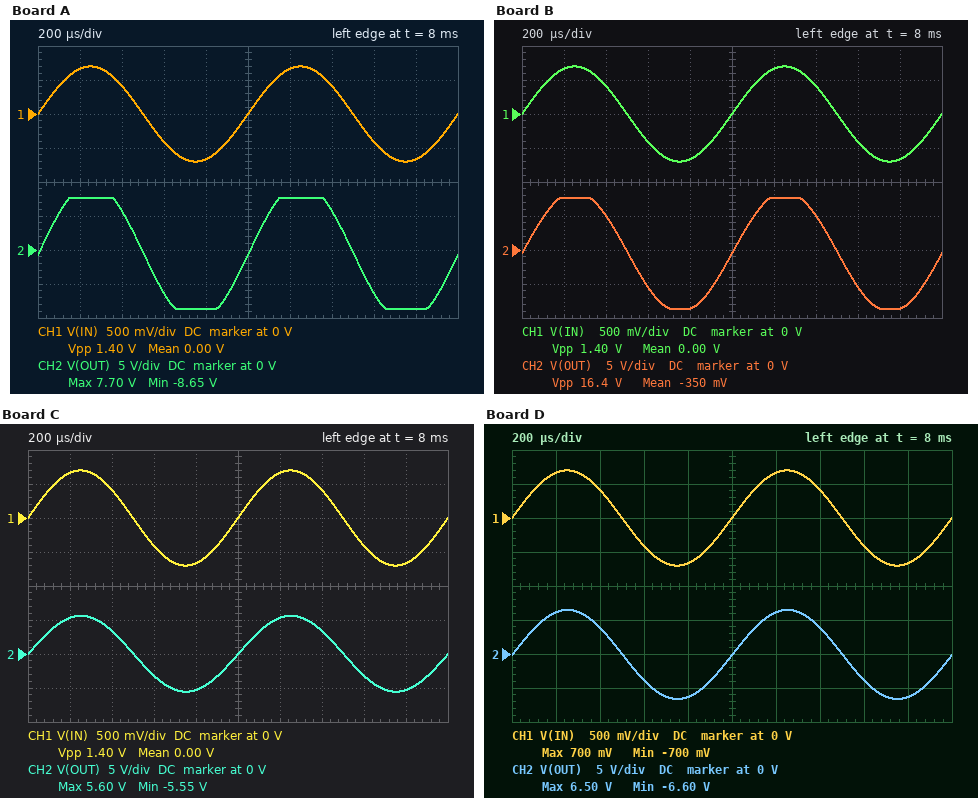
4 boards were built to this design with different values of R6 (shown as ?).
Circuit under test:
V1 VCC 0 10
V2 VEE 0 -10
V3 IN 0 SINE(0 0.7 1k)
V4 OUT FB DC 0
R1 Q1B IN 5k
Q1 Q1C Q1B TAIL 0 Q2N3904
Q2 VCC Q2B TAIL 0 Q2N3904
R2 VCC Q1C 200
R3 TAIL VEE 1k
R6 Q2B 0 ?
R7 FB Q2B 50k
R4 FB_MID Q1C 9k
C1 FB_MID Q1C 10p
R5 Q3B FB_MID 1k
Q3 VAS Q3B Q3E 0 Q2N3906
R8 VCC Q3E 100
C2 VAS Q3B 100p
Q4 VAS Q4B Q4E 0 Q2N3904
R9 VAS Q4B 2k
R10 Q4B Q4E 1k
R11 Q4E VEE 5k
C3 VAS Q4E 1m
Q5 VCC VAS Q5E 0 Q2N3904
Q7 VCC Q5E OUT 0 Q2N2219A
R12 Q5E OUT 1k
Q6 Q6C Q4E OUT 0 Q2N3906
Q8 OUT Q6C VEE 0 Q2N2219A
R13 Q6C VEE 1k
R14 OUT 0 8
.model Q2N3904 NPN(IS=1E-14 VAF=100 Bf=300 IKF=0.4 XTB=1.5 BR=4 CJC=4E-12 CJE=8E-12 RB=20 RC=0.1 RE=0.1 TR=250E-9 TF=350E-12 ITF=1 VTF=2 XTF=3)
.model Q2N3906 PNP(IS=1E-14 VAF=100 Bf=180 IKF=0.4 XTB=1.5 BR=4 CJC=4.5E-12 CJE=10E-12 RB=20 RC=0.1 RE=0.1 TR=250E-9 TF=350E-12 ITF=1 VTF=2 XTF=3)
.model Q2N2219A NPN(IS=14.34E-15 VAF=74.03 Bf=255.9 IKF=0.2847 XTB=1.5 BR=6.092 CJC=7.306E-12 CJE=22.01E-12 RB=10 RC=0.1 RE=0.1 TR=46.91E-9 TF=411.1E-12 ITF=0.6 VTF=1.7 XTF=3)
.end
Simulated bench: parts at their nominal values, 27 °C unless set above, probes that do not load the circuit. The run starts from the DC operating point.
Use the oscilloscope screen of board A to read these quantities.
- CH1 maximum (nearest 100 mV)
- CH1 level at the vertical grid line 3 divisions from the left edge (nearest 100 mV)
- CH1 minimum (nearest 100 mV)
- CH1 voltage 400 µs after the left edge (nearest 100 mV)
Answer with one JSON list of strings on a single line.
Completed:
["700 mV", "-400 mV", "-700 mV", "400 mV"]
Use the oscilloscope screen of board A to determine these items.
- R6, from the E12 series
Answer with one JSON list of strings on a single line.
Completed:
["3.3 kΩ"]
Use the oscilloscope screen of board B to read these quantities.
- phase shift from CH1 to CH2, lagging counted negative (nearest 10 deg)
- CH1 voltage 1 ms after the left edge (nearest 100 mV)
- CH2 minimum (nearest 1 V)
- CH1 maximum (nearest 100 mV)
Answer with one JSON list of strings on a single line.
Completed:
["0 deg", "0 V", "-9 V", "700 mV"]
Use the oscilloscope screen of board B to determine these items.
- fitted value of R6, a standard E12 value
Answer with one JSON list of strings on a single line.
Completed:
["3.9 kΩ"]
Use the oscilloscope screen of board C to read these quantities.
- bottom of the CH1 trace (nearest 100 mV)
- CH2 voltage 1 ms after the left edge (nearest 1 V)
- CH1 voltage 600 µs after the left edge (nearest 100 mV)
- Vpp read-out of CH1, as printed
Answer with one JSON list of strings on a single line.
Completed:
["-700 mV", "0 V", "-400 mV", "1.40 V"]
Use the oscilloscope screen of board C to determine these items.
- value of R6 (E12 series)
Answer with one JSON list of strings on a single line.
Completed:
["6.8 kΩ"]
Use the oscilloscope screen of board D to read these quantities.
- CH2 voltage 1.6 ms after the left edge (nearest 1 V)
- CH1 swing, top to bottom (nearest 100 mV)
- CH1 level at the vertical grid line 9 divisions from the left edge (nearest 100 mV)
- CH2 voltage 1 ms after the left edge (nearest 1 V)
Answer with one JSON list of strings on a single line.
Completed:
["-4 V", "1.4 V", "-700 mV", "0 V"]
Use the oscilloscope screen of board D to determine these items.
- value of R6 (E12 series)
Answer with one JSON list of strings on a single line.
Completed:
["5.6 kΩ"]
